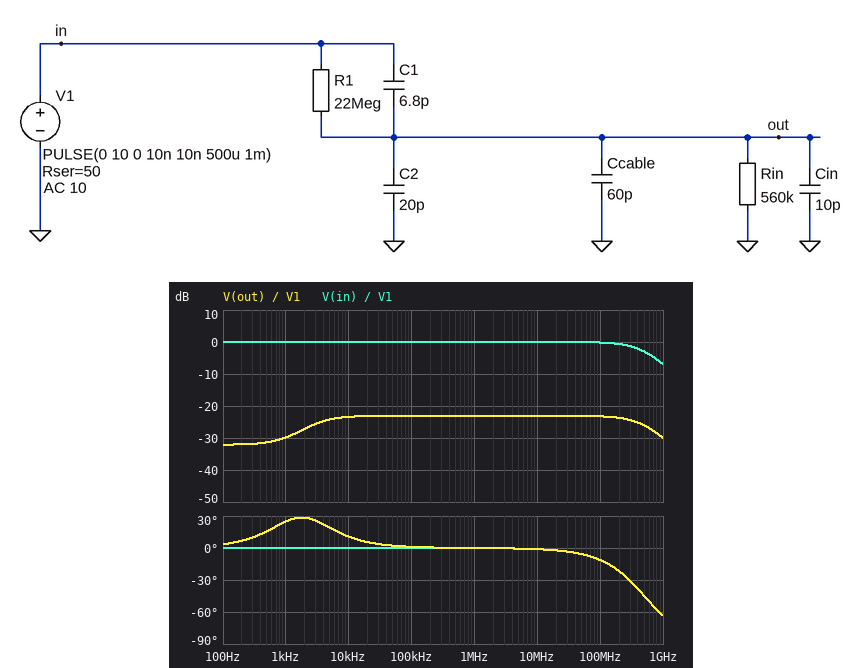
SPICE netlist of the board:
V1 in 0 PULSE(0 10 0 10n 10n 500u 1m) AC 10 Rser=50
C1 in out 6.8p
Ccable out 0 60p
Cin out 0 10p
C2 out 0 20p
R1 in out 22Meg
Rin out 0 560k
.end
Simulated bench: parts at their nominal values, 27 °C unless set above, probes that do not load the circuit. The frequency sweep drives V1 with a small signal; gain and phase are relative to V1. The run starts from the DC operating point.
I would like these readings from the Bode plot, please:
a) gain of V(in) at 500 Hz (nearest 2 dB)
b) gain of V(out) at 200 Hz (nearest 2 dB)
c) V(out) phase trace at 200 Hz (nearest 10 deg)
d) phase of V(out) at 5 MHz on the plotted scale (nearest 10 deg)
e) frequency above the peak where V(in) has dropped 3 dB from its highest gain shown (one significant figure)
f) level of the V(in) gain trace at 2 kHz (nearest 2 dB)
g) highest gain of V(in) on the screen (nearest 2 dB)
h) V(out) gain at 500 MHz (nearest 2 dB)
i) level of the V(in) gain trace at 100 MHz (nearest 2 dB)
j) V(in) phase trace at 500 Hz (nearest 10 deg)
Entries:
0 dB
-32 dB
10 deg
0 deg
500 MHz
0 dB
0 dB
-26 dB
0 dB
0 deg
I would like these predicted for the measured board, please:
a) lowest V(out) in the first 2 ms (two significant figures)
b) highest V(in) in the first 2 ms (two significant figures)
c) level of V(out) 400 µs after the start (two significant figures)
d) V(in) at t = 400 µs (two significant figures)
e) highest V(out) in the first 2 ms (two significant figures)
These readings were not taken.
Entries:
-450 mV
10 V
250 mV
10 V
700 mV
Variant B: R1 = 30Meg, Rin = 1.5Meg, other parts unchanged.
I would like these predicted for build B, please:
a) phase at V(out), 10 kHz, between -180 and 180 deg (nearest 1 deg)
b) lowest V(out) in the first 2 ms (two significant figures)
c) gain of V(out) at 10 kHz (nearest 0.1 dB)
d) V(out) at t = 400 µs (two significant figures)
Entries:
2 deg
-220 mV
-23.1 dB
490 mV
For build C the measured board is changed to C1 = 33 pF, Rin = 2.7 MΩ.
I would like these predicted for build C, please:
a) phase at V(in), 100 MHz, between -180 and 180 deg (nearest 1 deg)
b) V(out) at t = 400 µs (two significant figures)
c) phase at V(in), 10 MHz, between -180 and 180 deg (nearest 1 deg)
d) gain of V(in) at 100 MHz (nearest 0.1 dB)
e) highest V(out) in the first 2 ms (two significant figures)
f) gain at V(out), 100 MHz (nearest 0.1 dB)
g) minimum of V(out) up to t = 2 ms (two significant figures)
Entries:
-37 deg
1.5 V
-4 deg
-2.0 dB
2.7 V
-13.4 dB
-1.3 V
